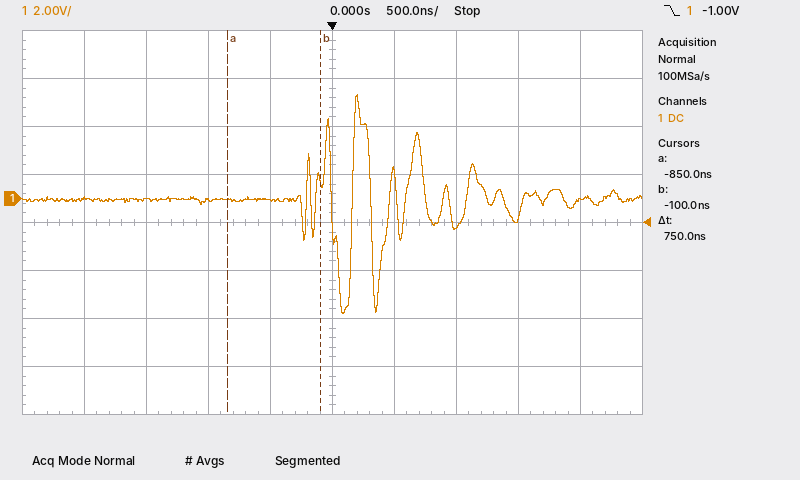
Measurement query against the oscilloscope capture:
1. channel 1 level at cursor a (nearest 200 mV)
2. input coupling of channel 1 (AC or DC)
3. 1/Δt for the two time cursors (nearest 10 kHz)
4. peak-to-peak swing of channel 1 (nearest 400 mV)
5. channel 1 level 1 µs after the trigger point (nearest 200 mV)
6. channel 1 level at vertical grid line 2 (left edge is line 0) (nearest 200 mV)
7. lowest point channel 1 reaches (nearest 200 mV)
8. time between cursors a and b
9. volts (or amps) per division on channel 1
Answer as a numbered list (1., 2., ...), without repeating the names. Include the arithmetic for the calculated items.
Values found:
1. 0.0 V
2. DC
3. 1 / 750 ns ≈ 1.33 MHz
4. 9.2 V
5. -1.2 V
6. 0.0 V
7. -4.8 V
8. 750 ns
9. 2 V
